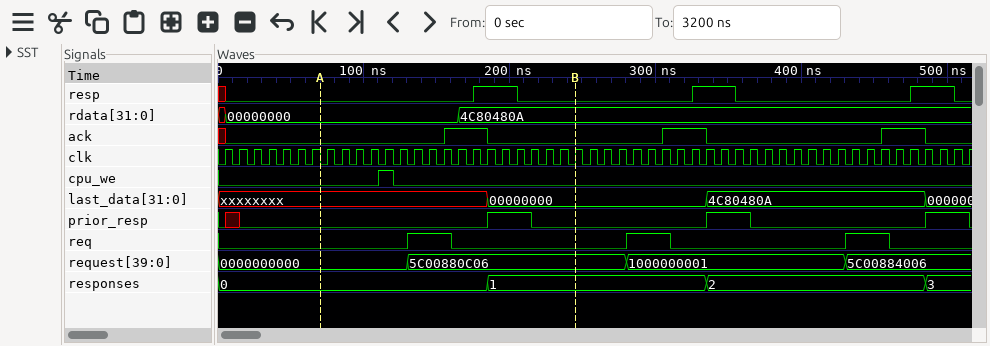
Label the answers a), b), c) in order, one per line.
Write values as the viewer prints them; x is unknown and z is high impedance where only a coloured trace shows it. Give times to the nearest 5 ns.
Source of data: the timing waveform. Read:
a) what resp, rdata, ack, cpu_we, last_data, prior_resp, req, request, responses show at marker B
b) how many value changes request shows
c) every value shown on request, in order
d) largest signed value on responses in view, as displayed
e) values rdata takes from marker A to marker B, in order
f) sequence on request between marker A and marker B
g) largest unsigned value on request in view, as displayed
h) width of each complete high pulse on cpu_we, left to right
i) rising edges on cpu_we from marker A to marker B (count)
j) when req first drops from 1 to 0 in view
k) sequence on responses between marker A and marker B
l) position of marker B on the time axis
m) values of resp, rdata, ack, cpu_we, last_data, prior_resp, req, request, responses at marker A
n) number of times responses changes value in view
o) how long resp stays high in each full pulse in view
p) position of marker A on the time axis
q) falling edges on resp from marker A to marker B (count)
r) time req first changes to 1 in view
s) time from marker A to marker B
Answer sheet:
a) resp=0, rdata=4C80480A, ack=0, cpu_we=0, last_data=00000000, prior_resp=0, req=0, request=5C00880C06, responses=1
b) 3
c) 0000000000, 5C00880C06, 1000000001, 5C00884006
d) 3
e) 00000000, 4C80480A
f) 0000000000, 5C00880C06
g) 5C00884006
h) 10 ns
i) 1
j) 160 ns
k) 0, 1
l) 245 ns
m) resp=0, rdata=00000000, ack=0, cpu_we=0, last_data=xxxxxxxx, prior_resp=0, req=0, request=0000000000, responses=0
n) 3
o) 30 ns, 30 ns, 30 ns
p) 70 ns
q) 1
r) 130 ns
s) 175 ns
